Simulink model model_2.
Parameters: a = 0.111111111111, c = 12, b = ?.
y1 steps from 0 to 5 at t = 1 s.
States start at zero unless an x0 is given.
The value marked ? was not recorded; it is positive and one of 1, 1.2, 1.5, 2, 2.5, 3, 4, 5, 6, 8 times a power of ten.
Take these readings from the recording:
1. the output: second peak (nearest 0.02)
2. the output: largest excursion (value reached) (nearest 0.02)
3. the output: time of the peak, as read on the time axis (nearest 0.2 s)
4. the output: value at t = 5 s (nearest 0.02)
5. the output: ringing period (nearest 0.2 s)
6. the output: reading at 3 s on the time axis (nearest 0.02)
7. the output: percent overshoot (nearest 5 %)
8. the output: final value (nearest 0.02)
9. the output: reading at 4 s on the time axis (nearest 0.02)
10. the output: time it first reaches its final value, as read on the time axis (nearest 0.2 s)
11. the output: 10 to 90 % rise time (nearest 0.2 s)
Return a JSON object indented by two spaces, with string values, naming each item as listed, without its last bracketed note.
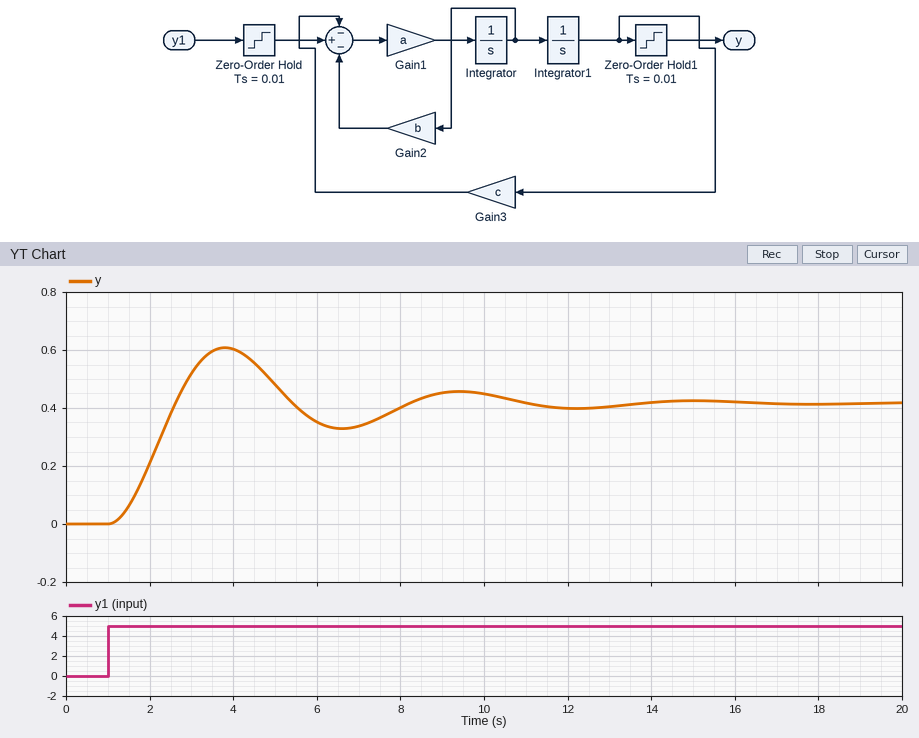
{
  "the output: second peak": "0.46",
  "the output: largest excursion (value reached)": "0.60",
  "the output: time of the peak, as read on the time axis": "3.8 s",
  "the output: value at t = 5 s": "0.48",
  "the output: ringing period": "5.6 s",
  "the output: reading at 3 s on the time axis": "0.52",
  "the output: percent overshoot": "45 %",
  "the output: final value": "0.42",
  "the output: reading at 4 s on the time axis": "0.60",
  "the output: time it first reaches its final value, as read on the time axis": "2.6 s",
  "the output: 10 to 90 % rise time": "1.0 s"
}
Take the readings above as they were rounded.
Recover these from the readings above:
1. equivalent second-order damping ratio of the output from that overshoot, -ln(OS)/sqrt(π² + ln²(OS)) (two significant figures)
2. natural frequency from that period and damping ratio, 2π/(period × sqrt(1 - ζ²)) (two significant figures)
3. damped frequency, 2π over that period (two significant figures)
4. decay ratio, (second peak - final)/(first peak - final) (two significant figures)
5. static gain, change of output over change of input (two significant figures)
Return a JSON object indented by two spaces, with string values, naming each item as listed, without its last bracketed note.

{
  "equivalent second-order damping ratio of the output from that overshoot, -ln(OS)/sqrt(π² + ln²(OS))": "0.25",
  "natural frequency from that period and damping ratio, 2π/(period × sqrt(1 - ζ²))": "1.2 rad/s",
  "damped frequency, 2π over that period": "1.1 rad/s",
  "decay ratio, (second peak - final)/(first peak - final)": "0.22",
  "static gain, change of output over change of input": "0.084"
}
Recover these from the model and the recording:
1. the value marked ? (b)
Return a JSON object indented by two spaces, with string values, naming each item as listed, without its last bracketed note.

{
  "the value marked ?": "5"
}
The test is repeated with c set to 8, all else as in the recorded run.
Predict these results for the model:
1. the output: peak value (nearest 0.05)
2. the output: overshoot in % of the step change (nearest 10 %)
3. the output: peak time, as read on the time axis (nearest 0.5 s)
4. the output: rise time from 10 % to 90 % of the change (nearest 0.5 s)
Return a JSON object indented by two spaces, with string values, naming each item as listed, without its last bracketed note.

{
  "the output: peak value": "0.85",
  "the output: overshoot in % of the step change": "40 %",
  "the output: peak time, as read on the time axis": "4.5 s",
  "the output: rise time from 10 % to 90 % of the change": "1.5 s"
}
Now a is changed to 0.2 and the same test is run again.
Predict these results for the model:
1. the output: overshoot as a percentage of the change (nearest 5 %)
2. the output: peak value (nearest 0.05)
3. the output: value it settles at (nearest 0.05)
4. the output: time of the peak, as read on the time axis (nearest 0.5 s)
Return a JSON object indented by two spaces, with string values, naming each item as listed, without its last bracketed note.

{
  "the output: overshoot as a percentage of the change": "35 %",
  "the output: peak value": "0.55",
  "the output: value it settles at": "0.40",
  "the output: time of the peak, as read on the time axis": "3.0 s"
}
